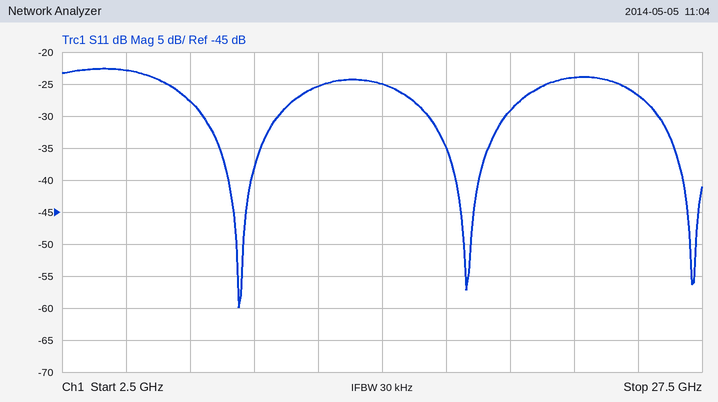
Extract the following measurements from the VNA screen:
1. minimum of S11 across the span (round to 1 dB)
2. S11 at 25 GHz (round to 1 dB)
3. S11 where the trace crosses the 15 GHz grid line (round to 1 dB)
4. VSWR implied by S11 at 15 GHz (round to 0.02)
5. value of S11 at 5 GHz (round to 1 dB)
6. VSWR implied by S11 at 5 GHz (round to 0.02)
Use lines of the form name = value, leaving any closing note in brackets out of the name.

minimum of S11 across the span = -60 dB
S11 at 25 GHz = -27 dB
S11 where the trace crosses the 15 GHz grid line = -25 dB
VSWR implied by S11 at 15 GHz = 1.12
value of S11 at 5 GHz = -23 dB
VSWR implied by S11 at 5 GHz = 1.16
